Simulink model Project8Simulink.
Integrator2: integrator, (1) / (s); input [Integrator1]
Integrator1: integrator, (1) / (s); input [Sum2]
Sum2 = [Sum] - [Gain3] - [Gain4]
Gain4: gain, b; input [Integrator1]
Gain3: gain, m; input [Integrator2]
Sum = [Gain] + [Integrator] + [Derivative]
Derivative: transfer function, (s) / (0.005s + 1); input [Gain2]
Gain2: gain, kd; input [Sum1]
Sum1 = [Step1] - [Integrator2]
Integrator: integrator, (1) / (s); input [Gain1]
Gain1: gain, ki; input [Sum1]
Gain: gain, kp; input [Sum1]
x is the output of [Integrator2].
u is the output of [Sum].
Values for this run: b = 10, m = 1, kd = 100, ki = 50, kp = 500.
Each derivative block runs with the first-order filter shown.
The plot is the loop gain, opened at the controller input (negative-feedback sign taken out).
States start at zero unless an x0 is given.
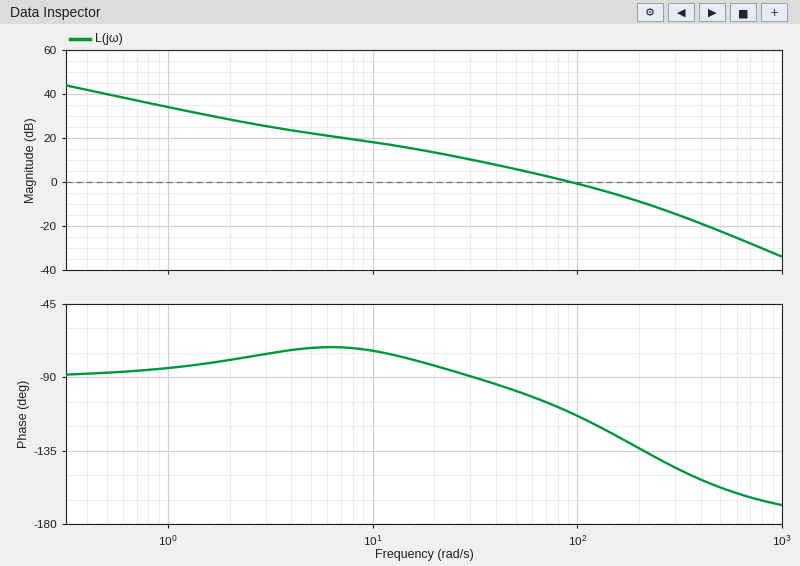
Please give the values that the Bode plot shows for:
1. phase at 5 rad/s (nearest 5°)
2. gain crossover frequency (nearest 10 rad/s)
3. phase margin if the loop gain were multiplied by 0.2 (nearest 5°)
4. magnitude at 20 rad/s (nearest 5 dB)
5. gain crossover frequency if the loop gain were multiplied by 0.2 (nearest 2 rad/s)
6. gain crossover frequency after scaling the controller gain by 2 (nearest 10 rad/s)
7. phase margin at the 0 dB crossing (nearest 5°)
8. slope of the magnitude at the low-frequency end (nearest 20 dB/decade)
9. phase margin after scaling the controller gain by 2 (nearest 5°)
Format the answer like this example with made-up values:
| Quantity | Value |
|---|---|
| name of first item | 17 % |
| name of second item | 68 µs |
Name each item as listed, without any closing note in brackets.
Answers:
| Quantity | Value |
|---|---|
| phase at 5 rad/s | -70° |
| gain crossover frequency | 90 rad/s |
| phase margin if the loop gain were multiplied by 0.2 | 100° |
| magnitude at 20 rad/s | 15 dB |
| gain crossover frequency if the loop gain were multiplied by 0.2 | 18 rad/s |
| gain crossover frequency after scaling the controller gain by 2 | 160 rad/s |
| phase margin at the 0 dB crossing | 70° |
| slope of the magnitude at the low-frequency end | -20 dB/decade |
| phase margin after scaling the controller gain by 2 | 55° |
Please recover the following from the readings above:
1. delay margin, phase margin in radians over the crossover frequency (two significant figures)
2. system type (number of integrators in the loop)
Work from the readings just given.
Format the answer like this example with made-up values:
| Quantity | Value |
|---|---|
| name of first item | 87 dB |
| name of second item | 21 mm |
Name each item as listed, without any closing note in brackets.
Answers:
| Quantity | Value |
|---|---|
| delay margin, phase margin in radians over the crossover frequency | 0.014 s |
| system type | 1 |
